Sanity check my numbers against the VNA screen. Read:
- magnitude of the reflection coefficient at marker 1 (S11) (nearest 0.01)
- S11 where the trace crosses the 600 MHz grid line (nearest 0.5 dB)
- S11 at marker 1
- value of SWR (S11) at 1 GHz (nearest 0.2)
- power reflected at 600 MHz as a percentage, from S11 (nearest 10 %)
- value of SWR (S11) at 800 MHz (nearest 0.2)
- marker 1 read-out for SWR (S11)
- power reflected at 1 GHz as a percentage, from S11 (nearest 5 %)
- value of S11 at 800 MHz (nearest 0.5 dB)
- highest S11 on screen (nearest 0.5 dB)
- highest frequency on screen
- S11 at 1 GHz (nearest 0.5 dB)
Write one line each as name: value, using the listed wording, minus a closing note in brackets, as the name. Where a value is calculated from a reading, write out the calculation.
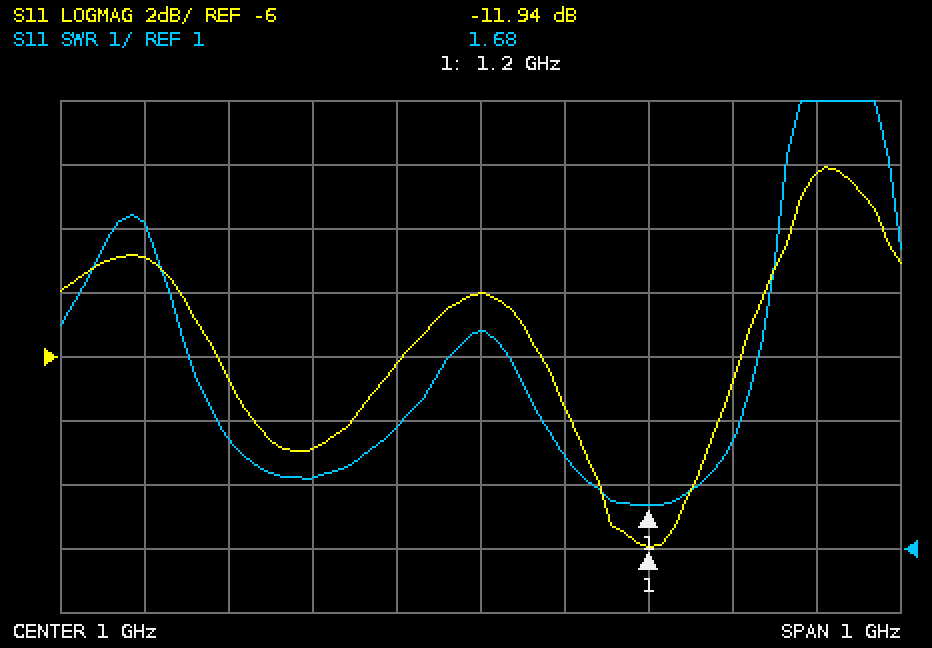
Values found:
magnitude of the reflection coefficient at marker 1 (S11): 10^(-11.94/20) ≈ 0.25
S11 where the trace crosses the 600 MHz grid line: -3.0 dB
S11 at marker 1: -11.94 dB
value of SWR (S11) at 1 GHz: 4.4
power reflected at 600 MHz as a percentage, from S11: 10^(-3/10) ≈ 50 %
value of SWR (S11) at 800 MHz: 2.2
marker 1 read-out for SWR: 1.68
power reflected at 1 GHz as a percentage, from S11: 10^(-4/10) ≈ 40 %
value of S11 at 800 MHz: -9.0 dB
highest S11 on screen: 0.0 dB
highest frequency on screen: 1.5 GHz
S11 at 1 GHz: -4.0 dB
